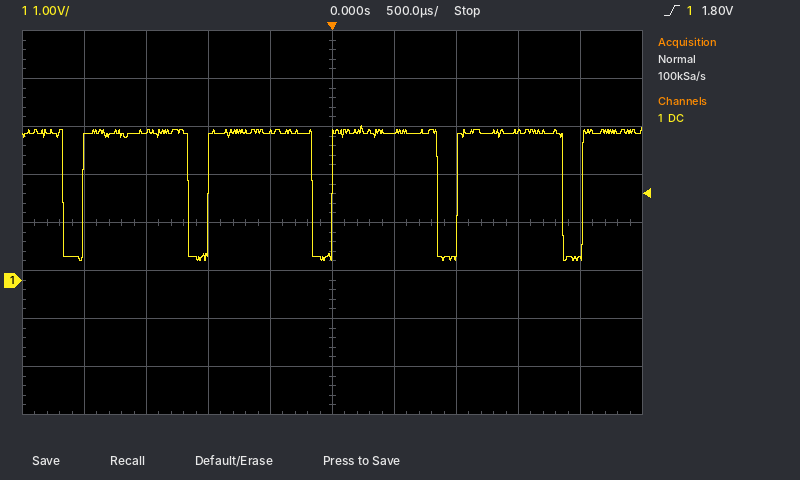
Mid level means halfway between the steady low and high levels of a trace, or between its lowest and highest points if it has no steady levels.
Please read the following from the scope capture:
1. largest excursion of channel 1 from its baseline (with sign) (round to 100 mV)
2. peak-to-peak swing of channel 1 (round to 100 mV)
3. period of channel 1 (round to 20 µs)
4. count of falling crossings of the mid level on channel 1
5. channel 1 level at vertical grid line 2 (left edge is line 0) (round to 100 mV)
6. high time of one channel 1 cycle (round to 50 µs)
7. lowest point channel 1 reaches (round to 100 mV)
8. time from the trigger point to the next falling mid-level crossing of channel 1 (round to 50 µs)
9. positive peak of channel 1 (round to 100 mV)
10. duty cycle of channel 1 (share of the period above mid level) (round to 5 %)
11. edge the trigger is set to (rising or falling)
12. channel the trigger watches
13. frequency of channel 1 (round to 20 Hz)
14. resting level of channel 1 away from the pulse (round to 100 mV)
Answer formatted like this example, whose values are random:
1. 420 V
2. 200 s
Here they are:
1. -2.7 V
2. 2.8 V
3. 1.00 ms
4. 5
5. 3.1 V
6. 850 µs
7. 400 mV
8. 850 µs
9. 3.2 V
10. 85 %
11. rising
12. channel 1
13. 1.00 kHz
14. 3.1 V
